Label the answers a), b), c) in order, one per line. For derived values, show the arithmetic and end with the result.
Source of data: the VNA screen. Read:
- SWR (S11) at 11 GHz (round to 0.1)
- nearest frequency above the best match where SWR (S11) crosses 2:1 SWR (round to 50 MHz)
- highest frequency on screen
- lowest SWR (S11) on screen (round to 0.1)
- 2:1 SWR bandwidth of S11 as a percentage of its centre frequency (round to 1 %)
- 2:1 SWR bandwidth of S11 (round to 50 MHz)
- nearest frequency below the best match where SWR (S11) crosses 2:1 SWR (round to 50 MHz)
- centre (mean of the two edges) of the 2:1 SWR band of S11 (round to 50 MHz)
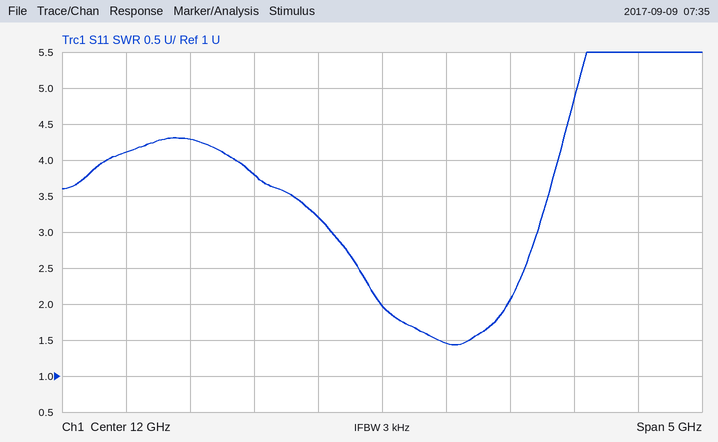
a) 3.8
b) 13.00 GHz
c) 14.5 GHz
d) 1.4
e) 1 GHz / 12.5 GHz ≈ 8 %
f) 13.00 GHz − 12.00 GHz = 1.00 GHz
g) 12.00 GHz
h) 12.50 GHz
